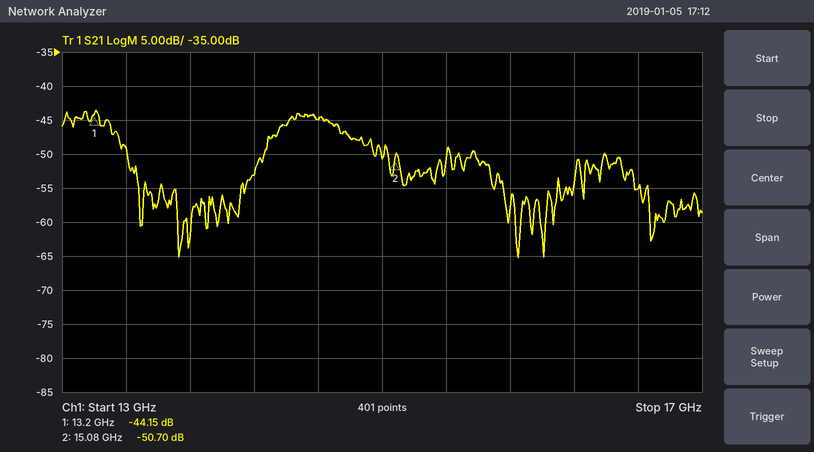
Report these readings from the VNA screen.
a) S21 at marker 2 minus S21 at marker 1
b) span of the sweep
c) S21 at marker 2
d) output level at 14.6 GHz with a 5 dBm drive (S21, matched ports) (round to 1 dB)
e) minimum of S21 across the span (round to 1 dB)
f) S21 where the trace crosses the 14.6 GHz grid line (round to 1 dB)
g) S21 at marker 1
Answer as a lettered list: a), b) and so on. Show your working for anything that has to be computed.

a) -50.7 − (-44.15) = -6.55 dB
b) 4 GHz
c) -50.70 dB
d) 5 dBm + (-45 dB) = -40 dBm
e) -65 dB
f) -45 dB
g) -44.15 dB
